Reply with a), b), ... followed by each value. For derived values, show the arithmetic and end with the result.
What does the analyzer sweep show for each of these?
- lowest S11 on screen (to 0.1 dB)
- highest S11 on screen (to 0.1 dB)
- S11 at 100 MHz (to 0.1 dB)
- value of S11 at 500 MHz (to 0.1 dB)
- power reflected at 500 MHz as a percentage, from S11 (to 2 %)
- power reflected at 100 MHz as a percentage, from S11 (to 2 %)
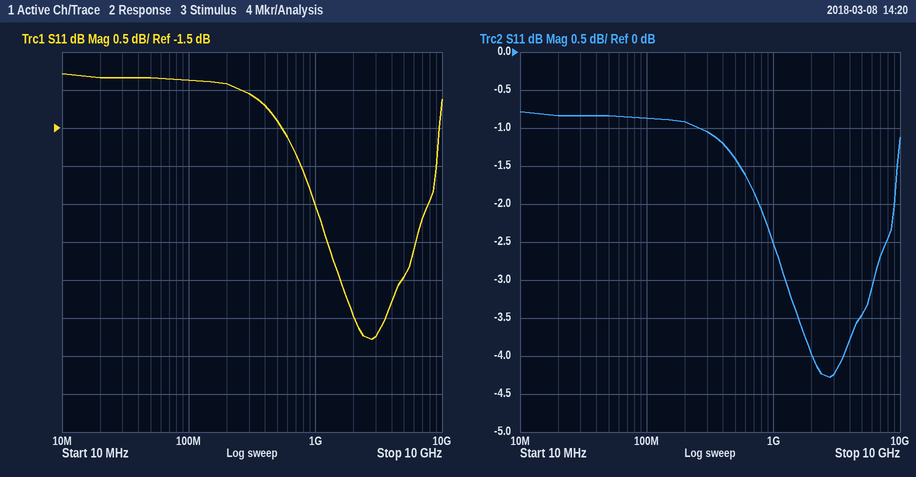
a) -4.3 dB
b) -0.8 dB
c) -0.9 dB
d) -1.4 dB
e) 10^(-1.4/10) ≈ 72 %
f) 10^(-0.9/10) ≈ 81.3 %, so 82 % to the nearest 2 %
